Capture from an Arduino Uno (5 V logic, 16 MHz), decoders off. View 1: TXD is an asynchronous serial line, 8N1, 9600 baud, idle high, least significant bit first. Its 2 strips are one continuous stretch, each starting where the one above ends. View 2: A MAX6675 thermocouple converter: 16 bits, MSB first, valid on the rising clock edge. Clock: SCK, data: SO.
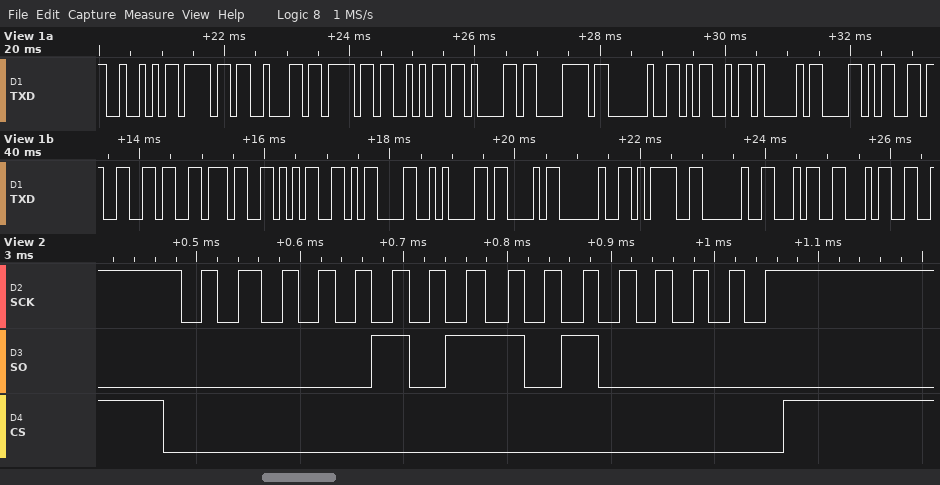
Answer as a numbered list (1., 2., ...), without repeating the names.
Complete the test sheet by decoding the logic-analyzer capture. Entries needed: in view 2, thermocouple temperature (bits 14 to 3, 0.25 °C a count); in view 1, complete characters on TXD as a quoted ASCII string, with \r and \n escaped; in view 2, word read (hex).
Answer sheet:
1. 45.00 °C
2. "Robojax MAX6675\r\nC = 44"
3. 0x05A0
